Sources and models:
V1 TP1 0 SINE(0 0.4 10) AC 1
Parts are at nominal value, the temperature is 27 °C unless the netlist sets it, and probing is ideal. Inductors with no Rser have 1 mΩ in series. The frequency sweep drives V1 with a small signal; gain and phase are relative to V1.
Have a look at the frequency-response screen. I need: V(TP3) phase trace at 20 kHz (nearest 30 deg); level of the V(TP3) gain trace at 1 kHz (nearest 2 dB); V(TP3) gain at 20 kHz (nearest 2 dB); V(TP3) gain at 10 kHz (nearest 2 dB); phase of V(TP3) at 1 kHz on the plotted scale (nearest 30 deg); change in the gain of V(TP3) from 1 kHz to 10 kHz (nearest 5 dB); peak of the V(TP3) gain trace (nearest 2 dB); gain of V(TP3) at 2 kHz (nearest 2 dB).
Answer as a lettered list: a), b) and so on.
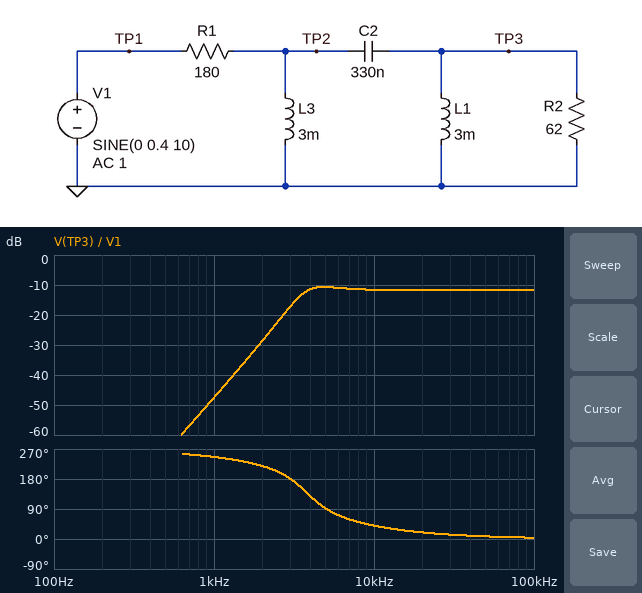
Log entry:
a) 30 deg
b) -48 dB
c) -12 dB
d) -12 dB
e) 240 deg
f) 35 dB
g) -10 dB
h) -28 dB
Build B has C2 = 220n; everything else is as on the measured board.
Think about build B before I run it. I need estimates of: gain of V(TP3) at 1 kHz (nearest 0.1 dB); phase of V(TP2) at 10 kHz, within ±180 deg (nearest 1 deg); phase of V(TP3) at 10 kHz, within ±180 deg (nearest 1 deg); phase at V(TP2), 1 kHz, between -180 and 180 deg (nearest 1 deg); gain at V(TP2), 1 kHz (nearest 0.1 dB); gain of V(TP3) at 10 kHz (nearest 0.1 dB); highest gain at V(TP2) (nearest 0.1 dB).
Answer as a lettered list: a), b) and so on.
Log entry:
a) -51.3 dB
b) -14 deg
c) 48 deg
d) 84 deg
e) -19.4 dB
f) -11.2 dB
g) -4.1 dB
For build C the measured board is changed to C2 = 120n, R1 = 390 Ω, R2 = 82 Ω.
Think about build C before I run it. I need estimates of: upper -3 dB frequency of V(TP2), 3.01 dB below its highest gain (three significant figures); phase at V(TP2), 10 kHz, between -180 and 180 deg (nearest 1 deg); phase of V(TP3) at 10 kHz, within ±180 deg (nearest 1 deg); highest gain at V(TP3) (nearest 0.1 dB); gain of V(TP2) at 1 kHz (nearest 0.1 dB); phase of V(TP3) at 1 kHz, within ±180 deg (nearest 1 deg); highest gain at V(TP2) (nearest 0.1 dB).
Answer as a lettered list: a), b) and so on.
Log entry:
a) 10.0 kHz
b) -11 deg
c) 68 deg
d) -12.8 dB
e) -26.2 dB
f) -106 deg
g) -6.0 dB
